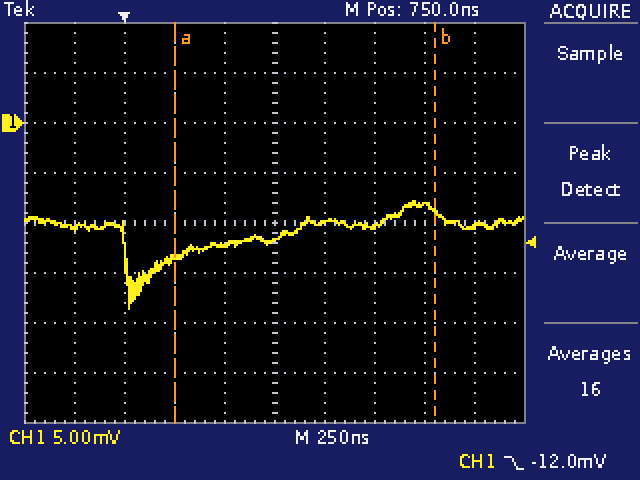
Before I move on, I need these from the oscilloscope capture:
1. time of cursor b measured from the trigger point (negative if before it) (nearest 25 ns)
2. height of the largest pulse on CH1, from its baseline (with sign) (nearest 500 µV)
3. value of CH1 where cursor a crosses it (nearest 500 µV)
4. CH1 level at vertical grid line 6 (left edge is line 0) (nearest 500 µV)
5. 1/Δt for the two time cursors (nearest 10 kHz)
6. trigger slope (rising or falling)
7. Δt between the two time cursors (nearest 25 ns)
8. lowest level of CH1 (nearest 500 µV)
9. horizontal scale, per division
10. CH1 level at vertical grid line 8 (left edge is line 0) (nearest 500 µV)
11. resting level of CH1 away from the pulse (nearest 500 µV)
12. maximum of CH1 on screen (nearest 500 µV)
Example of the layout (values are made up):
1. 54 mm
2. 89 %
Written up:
1. +1.550 µs
2. -8.5 mV
3. -13.5 mV
4. -10.0 mV
5. 770 kHz
6. falling
7. 1.300 µs
8. -18.5 mV
9. 250 ns
10. -8.0 mV
11. -10.0 mV
12. -8.0 mV
